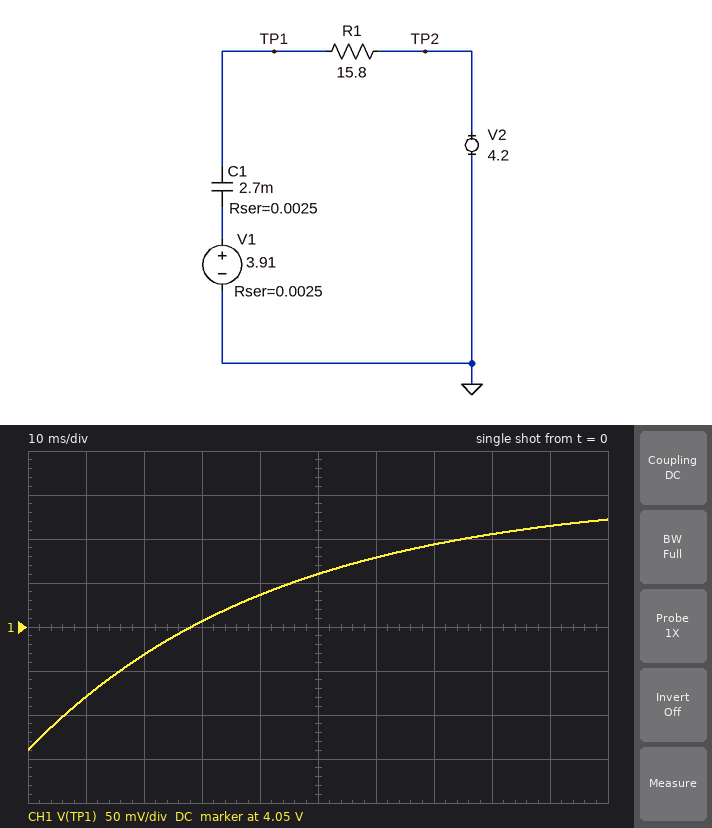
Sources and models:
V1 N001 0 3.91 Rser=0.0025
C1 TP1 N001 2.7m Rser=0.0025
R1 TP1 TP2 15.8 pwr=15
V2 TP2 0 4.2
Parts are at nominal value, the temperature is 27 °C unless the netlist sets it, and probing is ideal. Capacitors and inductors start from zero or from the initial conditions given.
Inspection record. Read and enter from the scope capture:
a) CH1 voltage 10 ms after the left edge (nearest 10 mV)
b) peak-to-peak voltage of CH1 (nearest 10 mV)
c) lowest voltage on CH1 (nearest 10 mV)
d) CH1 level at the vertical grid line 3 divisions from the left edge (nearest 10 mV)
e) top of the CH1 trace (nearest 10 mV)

3.97 V
260 mV
3.91 V
4.06 V
4.17 V
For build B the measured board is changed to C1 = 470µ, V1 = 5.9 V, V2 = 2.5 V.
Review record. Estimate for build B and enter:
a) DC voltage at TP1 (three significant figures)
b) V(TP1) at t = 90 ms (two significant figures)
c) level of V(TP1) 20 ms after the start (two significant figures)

2.50 V
2.5 V
2.7 V
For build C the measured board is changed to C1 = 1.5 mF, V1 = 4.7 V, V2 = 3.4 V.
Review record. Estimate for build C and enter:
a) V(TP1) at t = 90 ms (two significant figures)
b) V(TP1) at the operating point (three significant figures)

3.4 V
3.40 V
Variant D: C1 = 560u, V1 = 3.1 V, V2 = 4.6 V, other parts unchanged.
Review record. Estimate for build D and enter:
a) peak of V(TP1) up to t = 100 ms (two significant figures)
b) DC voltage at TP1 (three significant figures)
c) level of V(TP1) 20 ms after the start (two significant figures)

4.6 V
4.60 V
4.4 V
